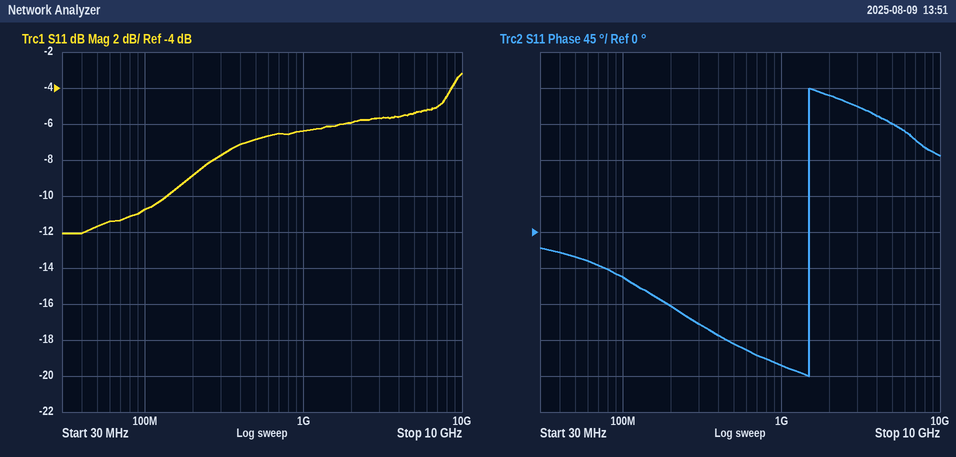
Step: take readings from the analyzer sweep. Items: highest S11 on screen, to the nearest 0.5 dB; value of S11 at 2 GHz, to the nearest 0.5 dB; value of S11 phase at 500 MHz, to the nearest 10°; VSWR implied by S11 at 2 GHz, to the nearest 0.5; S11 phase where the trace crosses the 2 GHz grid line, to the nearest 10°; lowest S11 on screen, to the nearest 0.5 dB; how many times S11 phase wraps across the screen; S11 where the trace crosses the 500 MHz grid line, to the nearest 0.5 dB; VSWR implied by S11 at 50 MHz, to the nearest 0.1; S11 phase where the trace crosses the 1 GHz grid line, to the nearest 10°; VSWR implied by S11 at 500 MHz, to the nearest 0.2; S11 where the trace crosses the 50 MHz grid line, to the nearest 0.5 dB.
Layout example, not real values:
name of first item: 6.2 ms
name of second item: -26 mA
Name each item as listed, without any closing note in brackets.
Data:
highest S11 on screen, to the nearest 0.5 dB: -3.0 dB
value of S11 at 2 GHz, to the nearest 0.5 dB: -6.0 dB
value of S11 phase at 500 MHz, to the nearest 10°: -140°
VSWR implied by S11 at 2 GHz, to the nearest 0.5: 3.0
S11 phase where the trace crosses the 2 GHz grid line, to the nearest 10°: 170°
lowest S11 on screen, to the nearest 0.5 dB: -12.0 dB
how many times S11 phase wraps across the screen: 1
S11 where the trace crosses the 500 MHz grid line, to the nearest 0.5 dB: -7.0 dB
VSWR implied by S11 at 50 MHz, to the nearest 0.1: 1.7
S11 phase where the trace crosses the 1 GHz grid line, to the nearest 10°: -170°
VSWR implied by S11 at 500 MHz, to the nearest 0.2: 2.6
S11 where the trace crosses the 50 MHz grid line, to the nearest 0.5 dB: -11.5 dB
